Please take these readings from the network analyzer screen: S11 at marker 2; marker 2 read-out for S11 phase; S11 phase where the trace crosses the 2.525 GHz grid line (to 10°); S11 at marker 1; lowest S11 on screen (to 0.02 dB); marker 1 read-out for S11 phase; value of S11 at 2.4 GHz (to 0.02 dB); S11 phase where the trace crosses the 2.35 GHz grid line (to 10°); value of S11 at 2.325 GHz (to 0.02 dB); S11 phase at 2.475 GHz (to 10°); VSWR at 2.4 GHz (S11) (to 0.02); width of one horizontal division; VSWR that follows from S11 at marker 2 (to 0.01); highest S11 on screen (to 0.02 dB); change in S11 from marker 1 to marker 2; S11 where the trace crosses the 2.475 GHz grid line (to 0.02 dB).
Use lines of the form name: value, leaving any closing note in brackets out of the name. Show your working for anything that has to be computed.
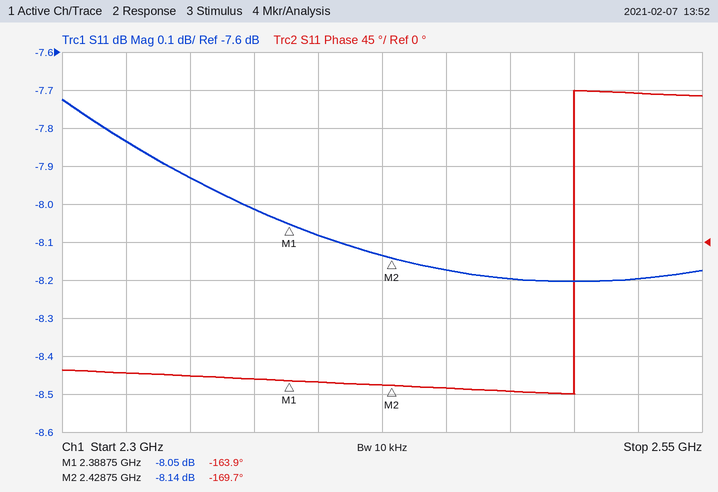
S11 at marker 2: -8.14 dB
marker 2 read-out for S11 phase: -169.7°
S11 phase where the trace crosses the 2.525 GHz grid line: 180°
S11 at marker 1: -8.05 dB
lowest S11 on screen: -8.20 dB
marker 1 read-out for S11 phase: -163.9°
value of S11 at 2.4 GHz: -8.08 dB
S11 phase where the trace crosses the 2.35 GHz grid line: -160°
value of S11 at 2.325 GHz: -7.84 dB
S11 phase at 2.475 GHz: -180°
VSWR at 2.4 GHz (S11): |Γ| = 10^(-8.08/20) = 0.3945; VSWR = (1 + 0.3945)/(1 − 0.3945) ≈ 2.30
width of one horizontal division: 25 MHz
VSWR that follows from S11 at marker 2: (1 + 0.3917)/(1 − 0.3917) ≈ 2.29
highest S11 on screen: -7.72 dB
change in S11 from marker 1 to marker 2: -8.14 − (-8.05) = -0.09 dB
S11 where the trace crosses the 2.475 GHz grid line: -8.20 dB
